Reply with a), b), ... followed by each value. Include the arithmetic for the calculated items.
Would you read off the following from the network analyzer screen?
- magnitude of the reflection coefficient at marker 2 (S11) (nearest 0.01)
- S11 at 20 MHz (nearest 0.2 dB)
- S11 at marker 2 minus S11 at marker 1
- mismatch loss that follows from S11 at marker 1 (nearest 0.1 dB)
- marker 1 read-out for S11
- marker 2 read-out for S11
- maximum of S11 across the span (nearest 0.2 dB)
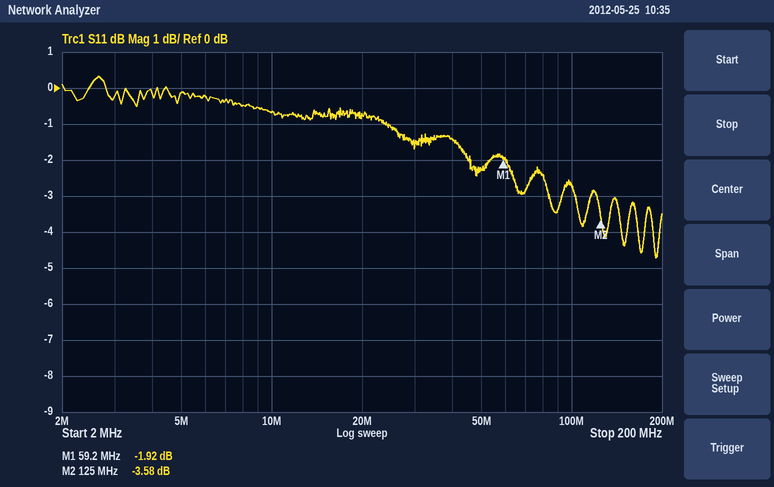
a) 10^(-3.58/20) ≈ 0.66
b) -0.8 dB
c) -3.58 − (-1.92) = -1.66 dB
d) −10 log10(1 − 10^(-1.92/10)) ≈ 4.5 dB
e) -1.92 dB
f) -3.58 dB
g) 0.4 dB
